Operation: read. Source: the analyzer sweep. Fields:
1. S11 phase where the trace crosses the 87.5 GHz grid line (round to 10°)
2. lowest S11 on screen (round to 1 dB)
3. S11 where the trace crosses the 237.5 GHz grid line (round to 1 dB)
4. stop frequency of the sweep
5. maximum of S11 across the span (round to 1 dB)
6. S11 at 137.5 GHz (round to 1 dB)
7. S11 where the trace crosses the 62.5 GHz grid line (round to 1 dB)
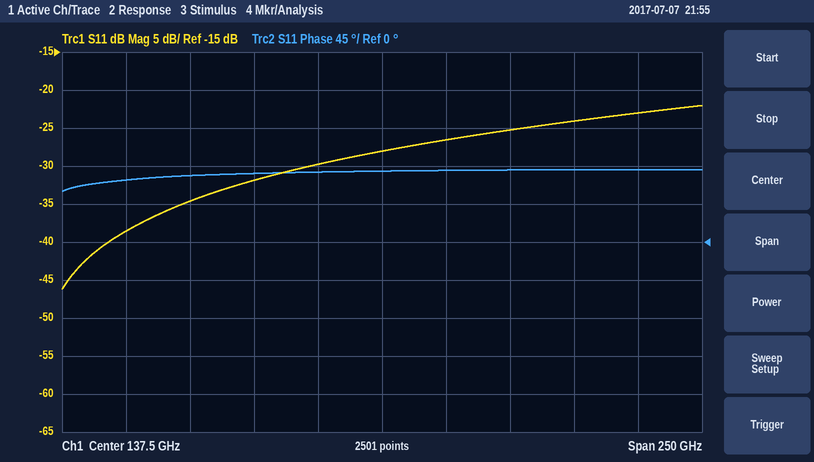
80°
-46 dB
-23 dB
262.5 GHz
-22 dB
-28 dB
-35 dB
